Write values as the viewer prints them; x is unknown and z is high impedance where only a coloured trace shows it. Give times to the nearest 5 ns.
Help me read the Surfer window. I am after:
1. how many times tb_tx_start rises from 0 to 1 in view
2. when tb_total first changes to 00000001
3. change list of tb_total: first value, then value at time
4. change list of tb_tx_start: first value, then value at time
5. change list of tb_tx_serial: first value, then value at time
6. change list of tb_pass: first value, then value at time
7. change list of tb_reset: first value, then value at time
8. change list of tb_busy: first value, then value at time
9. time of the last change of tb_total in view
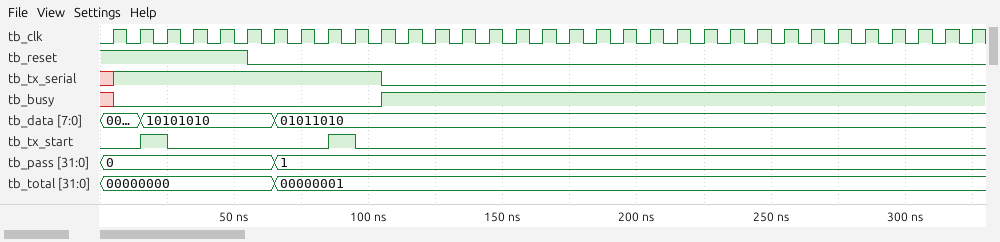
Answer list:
2
65 ns
00000000, 00000001 at 65 ns
0, 1 at 15 ns, 0 at 25 ns, 1 at 85 ns, 0 at 95 ns
x, 1 at 5 ns, 0 at 105 ns
0, 1 at 65 ns
1, 0 at 55 ns
x, 0 at 5 ns, 1 at 105 ns
65 ns
